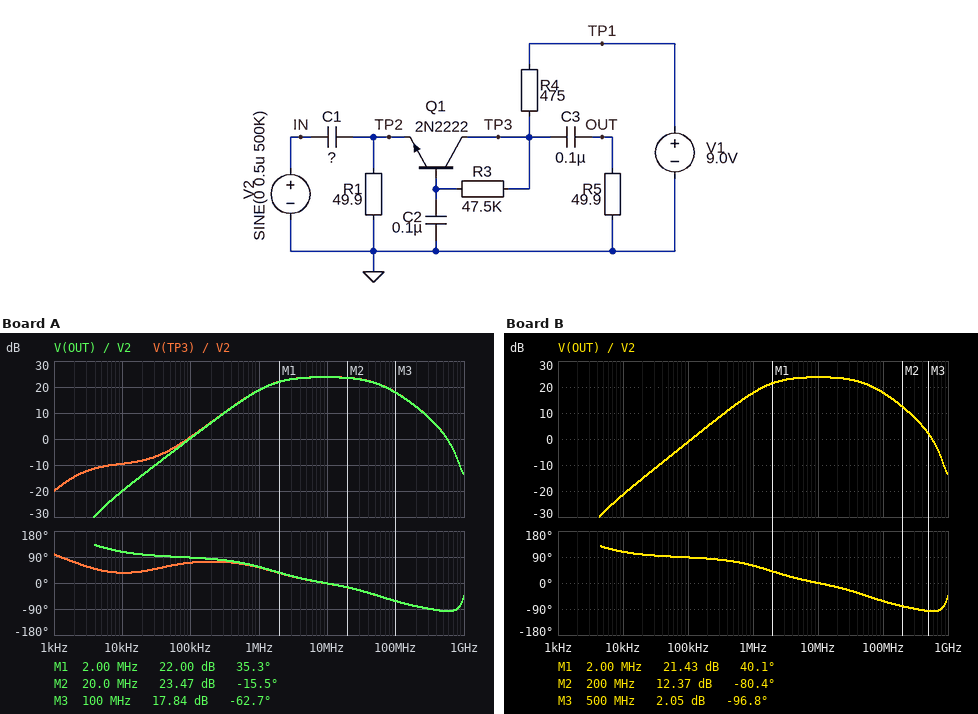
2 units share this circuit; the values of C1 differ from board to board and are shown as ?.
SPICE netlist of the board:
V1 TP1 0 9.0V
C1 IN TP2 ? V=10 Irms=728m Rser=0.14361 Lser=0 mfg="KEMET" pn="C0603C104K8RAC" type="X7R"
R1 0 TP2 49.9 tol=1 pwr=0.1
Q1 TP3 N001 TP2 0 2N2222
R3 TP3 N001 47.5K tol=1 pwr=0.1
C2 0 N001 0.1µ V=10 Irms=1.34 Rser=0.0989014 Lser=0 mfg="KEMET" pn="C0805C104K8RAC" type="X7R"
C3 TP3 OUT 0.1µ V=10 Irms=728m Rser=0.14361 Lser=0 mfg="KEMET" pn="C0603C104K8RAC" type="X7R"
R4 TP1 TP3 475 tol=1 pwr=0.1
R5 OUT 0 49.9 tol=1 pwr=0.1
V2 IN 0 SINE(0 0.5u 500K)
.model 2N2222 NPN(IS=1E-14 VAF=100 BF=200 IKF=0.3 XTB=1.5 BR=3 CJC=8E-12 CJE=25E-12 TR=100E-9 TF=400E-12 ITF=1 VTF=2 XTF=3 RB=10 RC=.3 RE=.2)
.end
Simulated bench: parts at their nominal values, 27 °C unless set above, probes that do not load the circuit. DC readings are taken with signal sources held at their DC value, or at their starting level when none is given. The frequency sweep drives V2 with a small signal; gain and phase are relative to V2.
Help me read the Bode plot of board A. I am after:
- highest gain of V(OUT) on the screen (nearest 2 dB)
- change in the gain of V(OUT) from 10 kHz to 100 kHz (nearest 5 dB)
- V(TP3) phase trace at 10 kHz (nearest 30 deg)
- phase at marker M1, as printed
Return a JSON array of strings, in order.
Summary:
["24 dB", "20 dB", "30 deg", "35.3 deg"]
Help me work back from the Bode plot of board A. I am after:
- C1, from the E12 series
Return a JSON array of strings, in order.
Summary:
["39 nF"]
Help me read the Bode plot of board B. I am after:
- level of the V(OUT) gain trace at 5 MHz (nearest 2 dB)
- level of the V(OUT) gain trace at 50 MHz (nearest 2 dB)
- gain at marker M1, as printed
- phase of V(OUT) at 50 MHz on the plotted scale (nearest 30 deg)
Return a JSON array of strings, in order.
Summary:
["24 dB", "22 dB", "21.43 dB", "-30 deg"]
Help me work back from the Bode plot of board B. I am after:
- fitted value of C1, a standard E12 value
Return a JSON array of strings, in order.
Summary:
["33 nF"]
